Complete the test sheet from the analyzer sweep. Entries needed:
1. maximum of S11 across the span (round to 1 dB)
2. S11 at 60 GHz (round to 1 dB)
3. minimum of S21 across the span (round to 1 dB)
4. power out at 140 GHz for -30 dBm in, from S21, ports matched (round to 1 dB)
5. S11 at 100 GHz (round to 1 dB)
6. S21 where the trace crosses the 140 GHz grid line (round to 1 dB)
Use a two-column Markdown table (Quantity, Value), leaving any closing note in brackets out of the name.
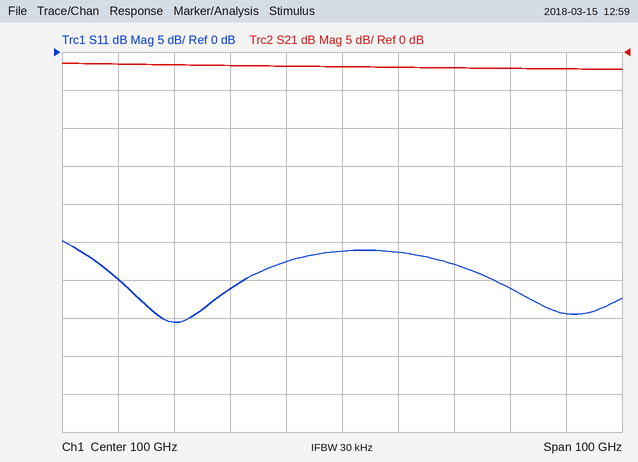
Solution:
| Quantity | Value |
|---|---|
| maximum of S11 across the span | -25 dB |
| S11 at 60 GHz | -30 dB |
| minimum of S21 across the span | -2 dB |
| power out at 140 GHz for -30 dBm in, from S21, ports matched | -32 dBm |
| S11 at 100 GHz | -26 dB |
| S21 where the trace crosses the 140 GHz grid line | -2 dB |
